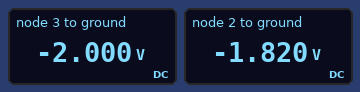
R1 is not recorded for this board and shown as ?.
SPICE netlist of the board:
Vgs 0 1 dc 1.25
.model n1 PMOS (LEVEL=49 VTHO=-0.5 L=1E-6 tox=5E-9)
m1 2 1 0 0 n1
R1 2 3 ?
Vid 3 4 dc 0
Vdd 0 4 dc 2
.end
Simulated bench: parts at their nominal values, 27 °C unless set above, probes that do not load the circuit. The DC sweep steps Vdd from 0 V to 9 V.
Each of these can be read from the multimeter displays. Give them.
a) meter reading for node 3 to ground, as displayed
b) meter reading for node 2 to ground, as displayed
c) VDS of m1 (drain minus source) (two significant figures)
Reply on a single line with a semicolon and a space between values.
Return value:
-2.000 V; -1.820 V; -1.8 V
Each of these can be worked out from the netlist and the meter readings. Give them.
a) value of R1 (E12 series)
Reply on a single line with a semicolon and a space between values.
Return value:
2.2 kΩ
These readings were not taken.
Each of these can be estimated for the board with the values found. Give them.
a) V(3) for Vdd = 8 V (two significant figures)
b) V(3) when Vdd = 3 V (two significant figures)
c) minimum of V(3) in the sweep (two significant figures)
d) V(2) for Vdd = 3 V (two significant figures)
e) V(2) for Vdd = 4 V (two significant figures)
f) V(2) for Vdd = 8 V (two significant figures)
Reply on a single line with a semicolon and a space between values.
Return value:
-8.0 V; -3.0 V; -9.0 V; -2.8 V; -3.8 V; -7.2 V
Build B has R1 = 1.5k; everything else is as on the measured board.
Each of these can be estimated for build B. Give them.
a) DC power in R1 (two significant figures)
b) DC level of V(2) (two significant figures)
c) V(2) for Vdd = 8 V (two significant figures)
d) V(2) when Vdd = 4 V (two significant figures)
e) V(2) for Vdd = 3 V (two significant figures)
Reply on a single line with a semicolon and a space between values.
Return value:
10 µW; -1.9 V; -7.4 V; -3.9 V; -2.9 V
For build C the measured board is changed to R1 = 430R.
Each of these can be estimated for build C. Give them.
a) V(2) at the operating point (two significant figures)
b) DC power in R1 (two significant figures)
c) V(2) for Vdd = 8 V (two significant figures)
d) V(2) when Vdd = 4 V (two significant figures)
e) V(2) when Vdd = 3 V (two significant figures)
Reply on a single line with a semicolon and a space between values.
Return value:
-2.0 V; 2.9 µW; -7.8 V; -4.0 V; -3.0 V
